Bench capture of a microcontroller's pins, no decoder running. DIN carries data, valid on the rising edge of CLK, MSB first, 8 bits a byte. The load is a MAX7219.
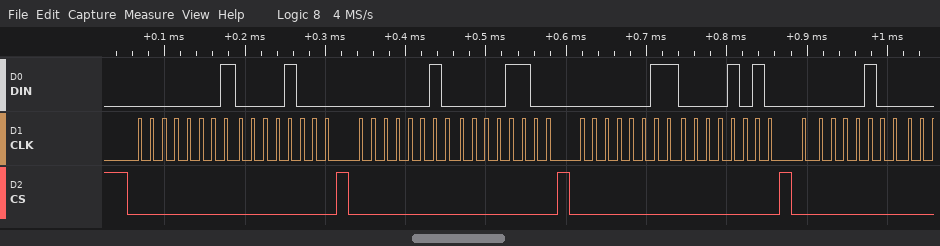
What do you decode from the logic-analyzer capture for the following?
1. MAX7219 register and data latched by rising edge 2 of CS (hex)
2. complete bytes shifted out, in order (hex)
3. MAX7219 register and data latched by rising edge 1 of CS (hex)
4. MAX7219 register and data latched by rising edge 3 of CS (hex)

register 0x2, data 0x0C
01 08 02 0C 03 0A 04
register 0x1, data 0x08
register 0x3, data 0x0A
